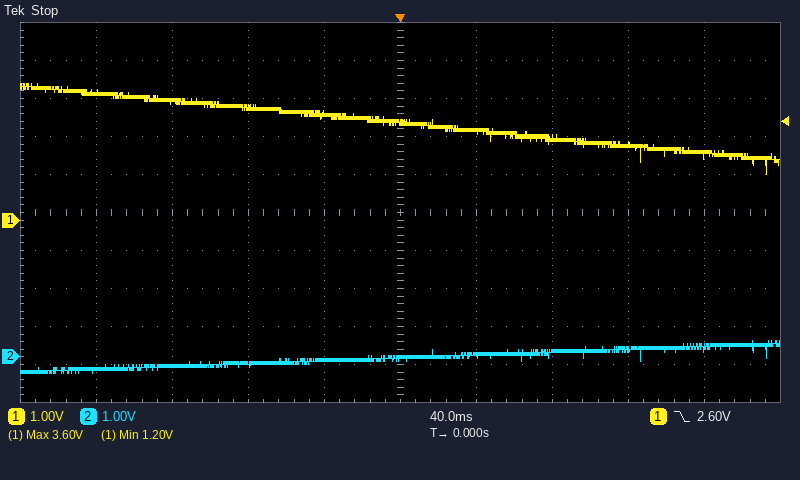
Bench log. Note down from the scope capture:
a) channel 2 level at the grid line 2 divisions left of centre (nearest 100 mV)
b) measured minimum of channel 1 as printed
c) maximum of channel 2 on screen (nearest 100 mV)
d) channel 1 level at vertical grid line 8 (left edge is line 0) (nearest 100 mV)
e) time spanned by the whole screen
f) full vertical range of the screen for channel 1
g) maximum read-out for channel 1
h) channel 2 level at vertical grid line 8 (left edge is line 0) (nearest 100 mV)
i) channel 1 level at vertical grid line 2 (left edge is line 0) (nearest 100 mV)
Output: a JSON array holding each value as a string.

["-200 mV", "1.20 V", "400 mV", "2.0 V", "400 ms", "10 V", "3.60 V", "200 mV", "3.1 V"]
